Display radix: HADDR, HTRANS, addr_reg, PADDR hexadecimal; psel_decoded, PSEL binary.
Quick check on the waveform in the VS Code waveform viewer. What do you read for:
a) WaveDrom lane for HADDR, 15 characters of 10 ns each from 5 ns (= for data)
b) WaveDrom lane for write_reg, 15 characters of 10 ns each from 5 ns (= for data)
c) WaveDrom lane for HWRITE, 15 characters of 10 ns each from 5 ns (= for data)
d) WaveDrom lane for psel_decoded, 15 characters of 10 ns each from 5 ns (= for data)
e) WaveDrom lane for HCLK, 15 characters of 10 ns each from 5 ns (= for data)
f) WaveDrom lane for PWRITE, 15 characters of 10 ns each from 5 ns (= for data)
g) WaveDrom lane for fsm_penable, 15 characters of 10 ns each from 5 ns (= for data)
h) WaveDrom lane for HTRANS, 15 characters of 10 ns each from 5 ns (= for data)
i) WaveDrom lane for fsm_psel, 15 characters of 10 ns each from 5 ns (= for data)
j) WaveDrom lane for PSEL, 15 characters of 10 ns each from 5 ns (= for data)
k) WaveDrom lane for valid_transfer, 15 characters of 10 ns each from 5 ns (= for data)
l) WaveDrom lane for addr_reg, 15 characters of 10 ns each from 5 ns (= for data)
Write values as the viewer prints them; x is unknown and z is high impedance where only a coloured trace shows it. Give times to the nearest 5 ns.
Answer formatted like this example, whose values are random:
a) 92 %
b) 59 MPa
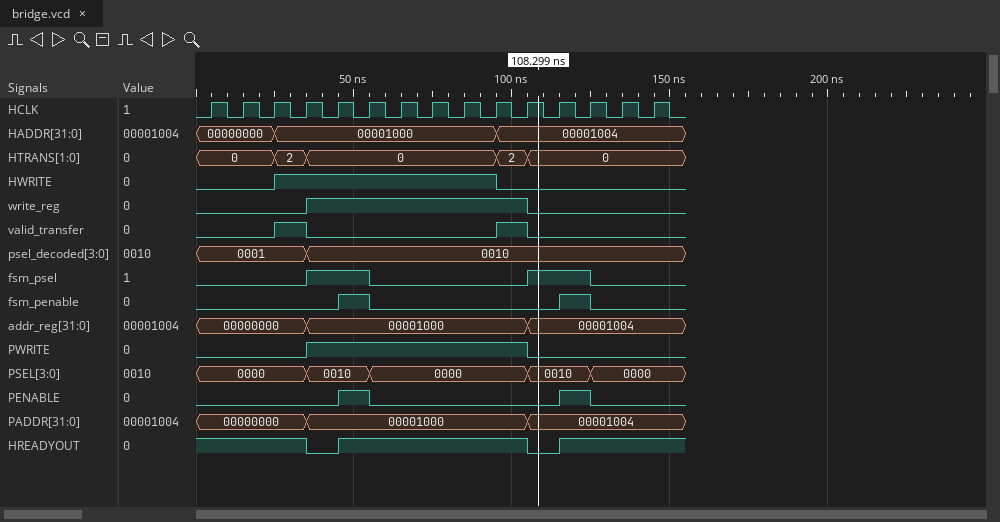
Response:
a) {name: 'HADDR', wave: '=.=......=.....', data: '00000000 00001000 00001004'}
b) {name: 'write_reg', wave: '0..1......0....'}
c) {name: 'HWRITE', wave: '0.1......0.....'}
d) {name: 'psel_decoded', wave: '=..=...........', data: '0001 0010'}
e) {name: 'HCLK', wave: 'p..............'}
f) {name: 'PWRITE', wave: '0..1......0....'}
g) {name: 'fsm_penable', wave: '0...10.....10..'}
h) {name: 'HTRANS', wave: '=.==.....==....', data: '0 2 0 2 0'}
i) {name: 'fsm_psel', wave: '0..1.0....1.0..'}
j) {name: 'PSEL', wave: '=..=.=....=.=..', data: '0000 0010 0000 0010 0000'}
k) {name: 'valid_transfer', wave: '0.10.....10....'}
l) {name: 'addr_reg', wave: '=..=......=....', data: '00000000 00001000 00001004'}
